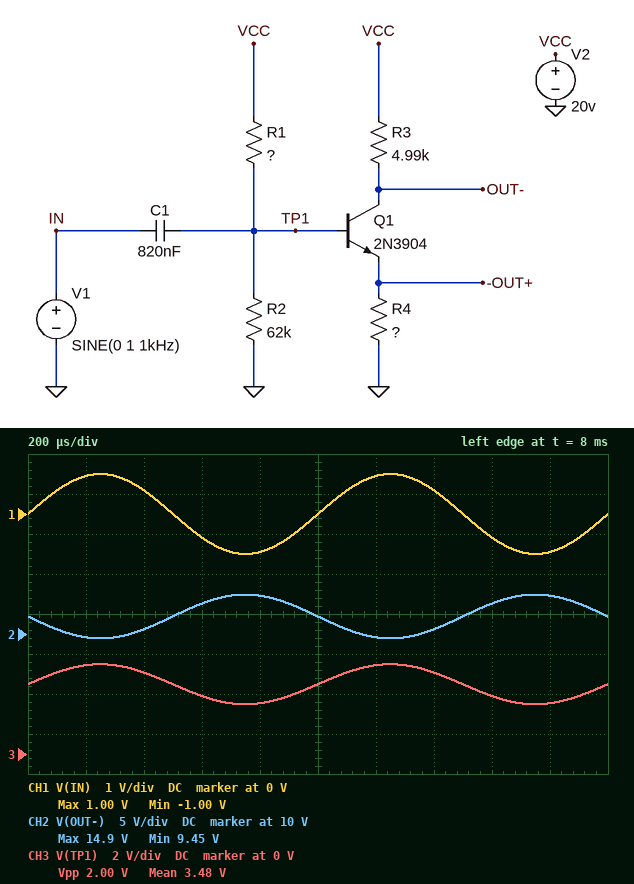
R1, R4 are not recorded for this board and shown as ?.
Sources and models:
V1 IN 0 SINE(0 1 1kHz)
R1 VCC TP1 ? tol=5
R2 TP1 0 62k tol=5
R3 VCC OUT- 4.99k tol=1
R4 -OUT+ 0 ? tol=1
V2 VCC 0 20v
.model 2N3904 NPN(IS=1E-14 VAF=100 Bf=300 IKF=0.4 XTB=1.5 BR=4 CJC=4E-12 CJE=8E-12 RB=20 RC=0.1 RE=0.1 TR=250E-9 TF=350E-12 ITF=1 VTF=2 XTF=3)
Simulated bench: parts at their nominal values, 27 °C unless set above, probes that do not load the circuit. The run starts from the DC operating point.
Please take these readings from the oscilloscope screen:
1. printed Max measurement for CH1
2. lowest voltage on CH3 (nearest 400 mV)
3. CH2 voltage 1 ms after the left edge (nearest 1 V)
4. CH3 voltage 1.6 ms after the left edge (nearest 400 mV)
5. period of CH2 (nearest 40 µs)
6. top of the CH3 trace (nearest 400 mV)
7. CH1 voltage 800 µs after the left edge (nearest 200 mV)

1.00 V
2.4 V
12 V
2.8 V
1.00 ms
4.4 V
-1.0 V
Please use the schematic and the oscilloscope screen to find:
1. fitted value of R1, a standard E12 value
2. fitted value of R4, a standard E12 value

270 kΩ
1.8 kΩ
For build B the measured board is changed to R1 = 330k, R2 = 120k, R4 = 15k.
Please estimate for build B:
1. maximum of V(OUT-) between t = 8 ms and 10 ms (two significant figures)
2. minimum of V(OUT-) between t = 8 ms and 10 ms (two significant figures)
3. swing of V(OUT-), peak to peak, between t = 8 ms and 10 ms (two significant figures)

19 V
18 V
660 mV
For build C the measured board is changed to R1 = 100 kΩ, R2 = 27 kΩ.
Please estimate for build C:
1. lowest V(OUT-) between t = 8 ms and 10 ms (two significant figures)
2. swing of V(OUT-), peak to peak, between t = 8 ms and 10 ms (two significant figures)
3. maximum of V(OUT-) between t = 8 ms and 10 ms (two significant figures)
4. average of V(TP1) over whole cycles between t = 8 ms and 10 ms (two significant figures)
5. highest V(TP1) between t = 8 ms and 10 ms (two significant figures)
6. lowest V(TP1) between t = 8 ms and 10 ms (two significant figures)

7.7 V
5.5 V
13 V
4.1 V
5.1 V
3.1 V
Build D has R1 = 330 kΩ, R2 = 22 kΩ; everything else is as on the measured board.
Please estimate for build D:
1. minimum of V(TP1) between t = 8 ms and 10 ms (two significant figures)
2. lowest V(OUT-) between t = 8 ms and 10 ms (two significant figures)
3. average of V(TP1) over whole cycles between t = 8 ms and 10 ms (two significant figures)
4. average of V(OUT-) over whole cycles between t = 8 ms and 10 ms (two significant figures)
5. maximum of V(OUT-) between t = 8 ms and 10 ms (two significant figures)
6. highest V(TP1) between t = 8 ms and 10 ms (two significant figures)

220 mV
16 V
1.2 V
18 V
20 V
2.2 V
